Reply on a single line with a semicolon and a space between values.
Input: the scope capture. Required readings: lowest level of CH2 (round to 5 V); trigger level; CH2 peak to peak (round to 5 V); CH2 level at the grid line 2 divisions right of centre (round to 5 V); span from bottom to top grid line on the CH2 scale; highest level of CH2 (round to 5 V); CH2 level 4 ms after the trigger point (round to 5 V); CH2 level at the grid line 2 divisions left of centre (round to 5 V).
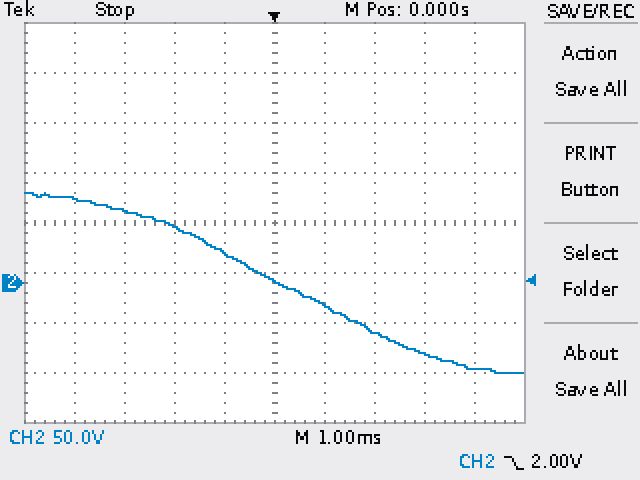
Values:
-90 V; 2.00 V; 180 V; -50 V; 400 V; 90 V; -85 V; 55 V
